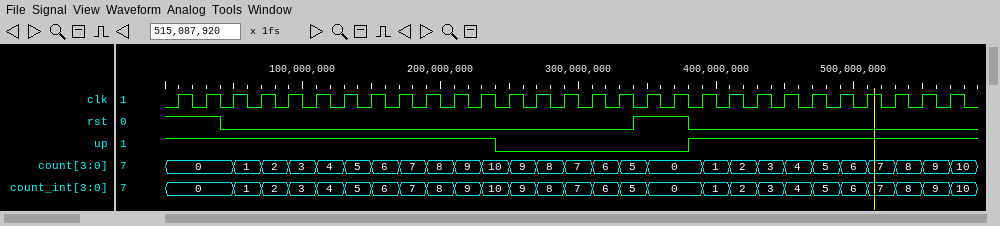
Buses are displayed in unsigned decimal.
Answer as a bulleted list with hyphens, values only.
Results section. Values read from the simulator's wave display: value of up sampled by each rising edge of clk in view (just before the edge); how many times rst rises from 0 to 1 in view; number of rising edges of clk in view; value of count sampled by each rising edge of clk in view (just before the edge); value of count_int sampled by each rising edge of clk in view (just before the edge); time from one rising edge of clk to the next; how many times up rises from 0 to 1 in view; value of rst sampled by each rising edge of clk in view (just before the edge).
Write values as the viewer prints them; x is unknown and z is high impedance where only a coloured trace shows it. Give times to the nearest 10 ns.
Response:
- 1 1 1 1 1 1 1 1 1 1 1 1 0 0 0 0 0 0 0 1 1 1 1 1 1 1 1 1 1
- 1
- 29
- 0, 0, 0, 1, 2, 3, 4, 5, 6, 7, 8, 9, 10, 9, 8, 7, 6, 5, 0, 0, 1, 2, 3, 4, 5, 6, 7, 8, 9
- 0, 0, 0, 1, 2, 3, 4, 5, 6, 7, 8, 9, 10, 9, 8, 7, 6, 5, 0, 0, 1, 2, 3, 4, 5, 6, 7, 8, 9
- 20 ns
- 1
- 1 1 0 0 0 0 0 0 0 0 0 0 0 0 0 0 0 1 1 0 0 0 0 0 0 0 0 0 0
